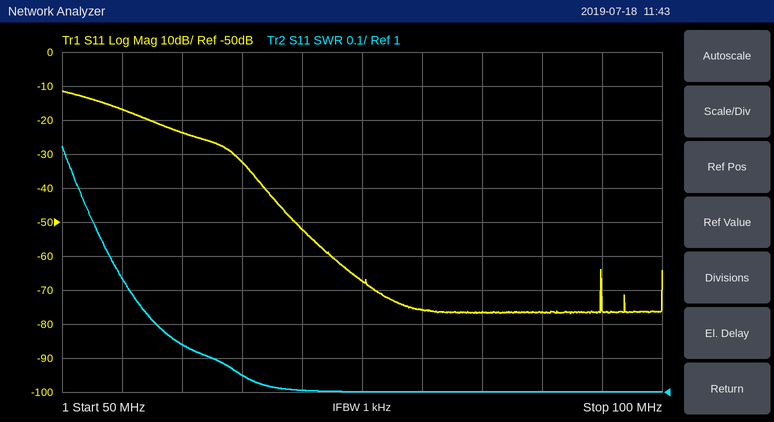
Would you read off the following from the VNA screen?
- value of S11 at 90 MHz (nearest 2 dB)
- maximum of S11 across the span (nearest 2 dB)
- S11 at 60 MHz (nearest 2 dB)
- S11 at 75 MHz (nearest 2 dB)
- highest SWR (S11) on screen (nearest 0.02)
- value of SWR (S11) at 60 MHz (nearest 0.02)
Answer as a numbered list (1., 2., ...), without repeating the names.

1. -76 dB
2. -12 dB
3. -24 dB
4. -68 dB
5. 1.72
6. 1.14
